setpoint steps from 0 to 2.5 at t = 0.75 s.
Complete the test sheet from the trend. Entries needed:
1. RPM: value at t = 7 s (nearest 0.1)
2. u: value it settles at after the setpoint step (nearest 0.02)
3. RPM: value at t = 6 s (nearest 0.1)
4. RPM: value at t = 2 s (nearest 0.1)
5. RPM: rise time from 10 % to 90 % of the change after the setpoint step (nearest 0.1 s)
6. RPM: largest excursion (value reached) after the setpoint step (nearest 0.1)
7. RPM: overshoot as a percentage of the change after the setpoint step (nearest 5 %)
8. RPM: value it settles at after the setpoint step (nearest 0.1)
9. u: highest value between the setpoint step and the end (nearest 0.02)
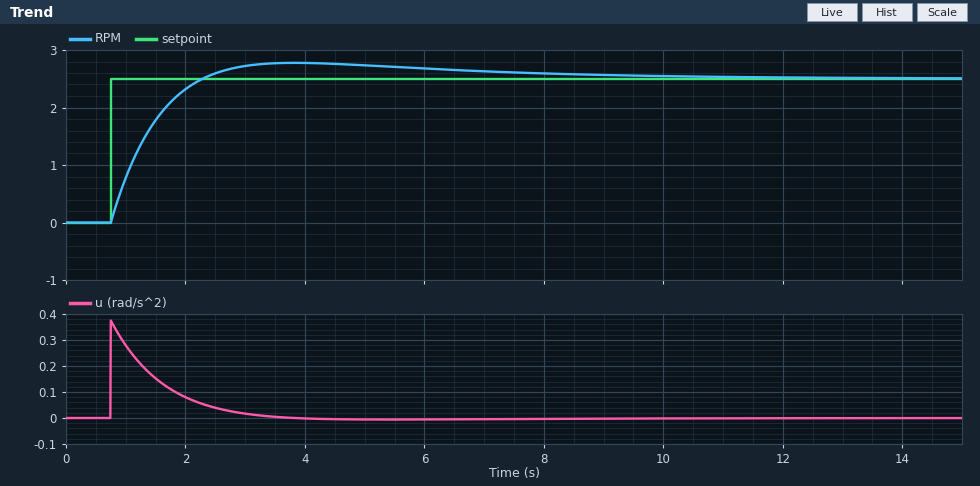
2.6
0.00
2.7
2.3
1.1 s
2.8
10 %
2.5
0.38
